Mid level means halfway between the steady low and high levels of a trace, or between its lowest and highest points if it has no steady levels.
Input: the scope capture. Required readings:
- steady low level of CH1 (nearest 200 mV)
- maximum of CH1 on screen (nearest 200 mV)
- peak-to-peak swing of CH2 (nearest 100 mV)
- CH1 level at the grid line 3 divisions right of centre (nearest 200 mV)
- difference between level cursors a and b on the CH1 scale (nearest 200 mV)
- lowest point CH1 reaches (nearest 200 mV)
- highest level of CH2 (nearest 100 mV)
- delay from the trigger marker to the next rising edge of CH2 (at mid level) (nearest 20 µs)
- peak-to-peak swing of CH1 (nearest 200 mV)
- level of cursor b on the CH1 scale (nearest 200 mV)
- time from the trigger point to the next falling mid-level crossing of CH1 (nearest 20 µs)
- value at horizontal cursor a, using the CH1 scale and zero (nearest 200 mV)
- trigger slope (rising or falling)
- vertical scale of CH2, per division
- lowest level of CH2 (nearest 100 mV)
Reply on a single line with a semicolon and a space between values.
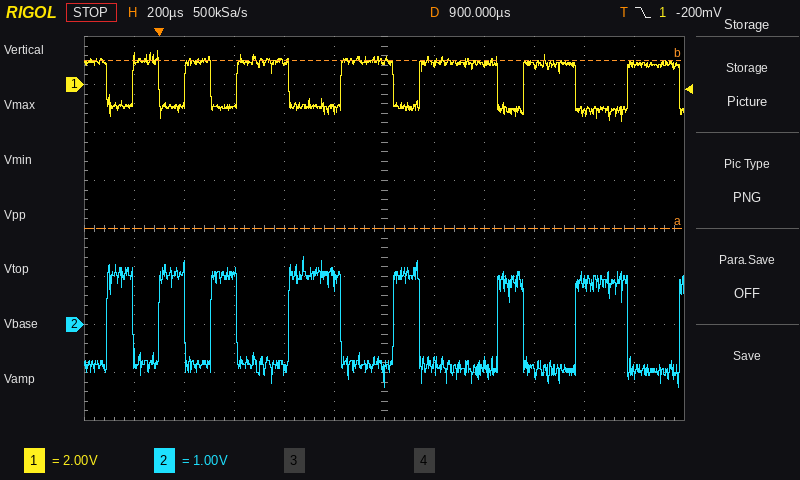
-1.0 V; 1.4 V; 2.7 V; 800 mV; 7.0 V; -1.6 V; 1.4 V; 200 µs; 3.0 V; 1.0 V; 200 µs; -6.0 V; falling; 1 V; -1.3 V
